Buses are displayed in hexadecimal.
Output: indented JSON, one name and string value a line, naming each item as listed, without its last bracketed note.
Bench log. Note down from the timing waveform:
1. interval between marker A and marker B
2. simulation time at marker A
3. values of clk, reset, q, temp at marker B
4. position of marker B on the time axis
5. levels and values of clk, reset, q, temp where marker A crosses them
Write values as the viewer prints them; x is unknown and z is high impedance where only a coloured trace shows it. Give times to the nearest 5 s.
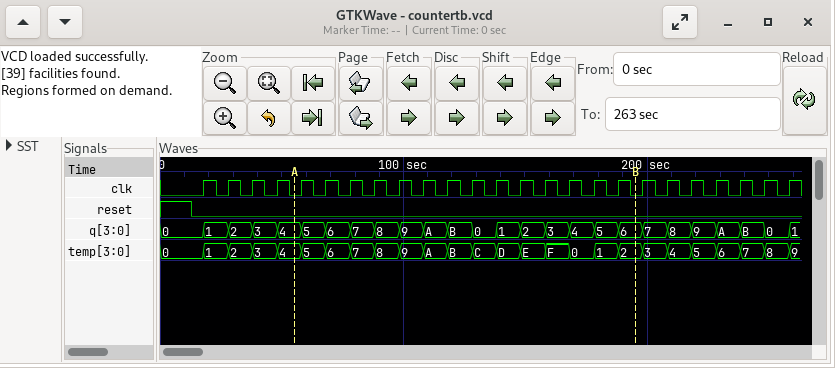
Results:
{
  "interval between marker A and marker B": "140 s",
  "simulation time at marker A": "55 s",
  "values of clk, reset, q, temp at marker B": "clk=0, reset=0, q=6, temp=2",
  "position of marker B on the time axis": "195 s",
  "levels and values of clk, reset, q, temp where marker A crosses them": "clk=0, reset=0, q=4, temp=4"
}
